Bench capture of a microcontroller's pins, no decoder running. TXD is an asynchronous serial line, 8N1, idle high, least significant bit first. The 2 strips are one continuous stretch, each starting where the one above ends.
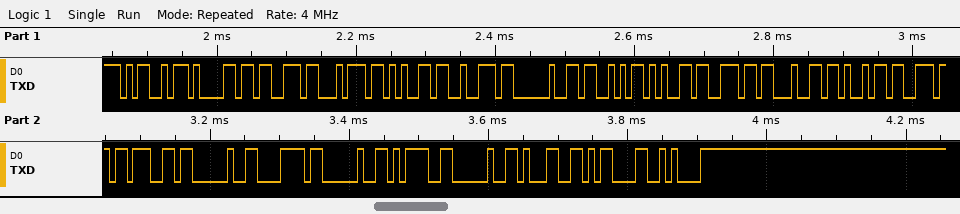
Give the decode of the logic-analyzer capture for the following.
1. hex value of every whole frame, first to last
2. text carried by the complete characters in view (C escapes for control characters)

4D 61 73 74 65 72 20 53 65 6E 64 69 6E 67 20 78 20 3D 20 31 0D 0A
"Master Sending x = 1\r\n"
